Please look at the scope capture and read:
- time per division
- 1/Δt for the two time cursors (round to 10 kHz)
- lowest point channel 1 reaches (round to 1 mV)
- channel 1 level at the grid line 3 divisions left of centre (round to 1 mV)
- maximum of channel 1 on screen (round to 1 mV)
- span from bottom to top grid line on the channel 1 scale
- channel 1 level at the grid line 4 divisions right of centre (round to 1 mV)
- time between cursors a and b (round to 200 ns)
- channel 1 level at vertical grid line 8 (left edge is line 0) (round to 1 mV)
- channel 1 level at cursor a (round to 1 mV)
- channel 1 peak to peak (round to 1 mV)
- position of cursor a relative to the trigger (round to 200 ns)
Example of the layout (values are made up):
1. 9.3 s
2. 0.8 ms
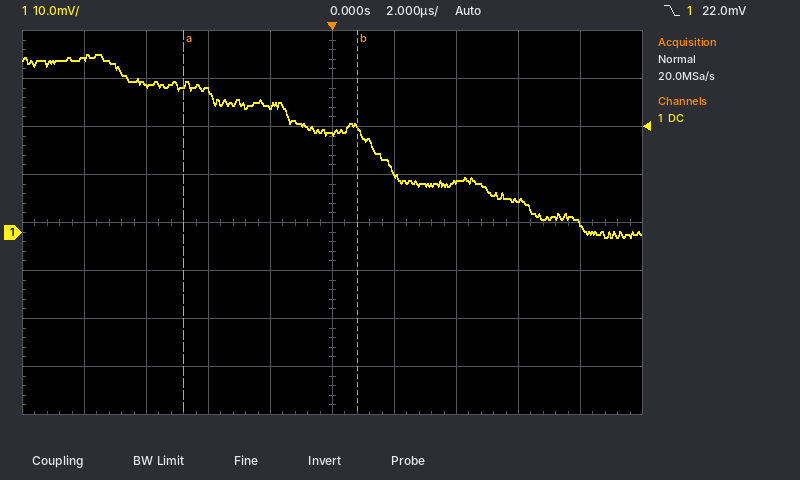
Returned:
1. 2 µs
2. 180 kHz
3. -1 mV
4. 31 mV
5. 37 mV
6. 80 mV
7. 2 mV
8. 5.6 µs
9. 7 mV
10. 31 mV
11. 38 mV
12. -4.8 µs
